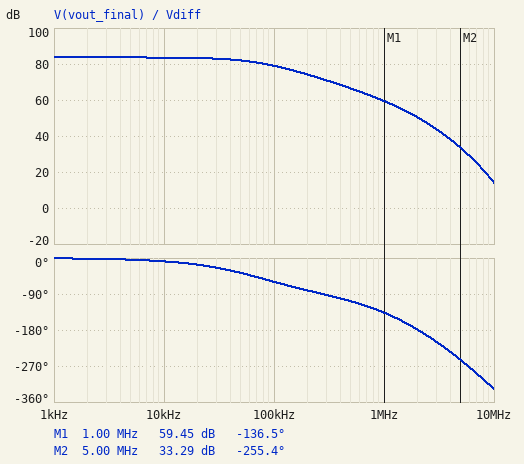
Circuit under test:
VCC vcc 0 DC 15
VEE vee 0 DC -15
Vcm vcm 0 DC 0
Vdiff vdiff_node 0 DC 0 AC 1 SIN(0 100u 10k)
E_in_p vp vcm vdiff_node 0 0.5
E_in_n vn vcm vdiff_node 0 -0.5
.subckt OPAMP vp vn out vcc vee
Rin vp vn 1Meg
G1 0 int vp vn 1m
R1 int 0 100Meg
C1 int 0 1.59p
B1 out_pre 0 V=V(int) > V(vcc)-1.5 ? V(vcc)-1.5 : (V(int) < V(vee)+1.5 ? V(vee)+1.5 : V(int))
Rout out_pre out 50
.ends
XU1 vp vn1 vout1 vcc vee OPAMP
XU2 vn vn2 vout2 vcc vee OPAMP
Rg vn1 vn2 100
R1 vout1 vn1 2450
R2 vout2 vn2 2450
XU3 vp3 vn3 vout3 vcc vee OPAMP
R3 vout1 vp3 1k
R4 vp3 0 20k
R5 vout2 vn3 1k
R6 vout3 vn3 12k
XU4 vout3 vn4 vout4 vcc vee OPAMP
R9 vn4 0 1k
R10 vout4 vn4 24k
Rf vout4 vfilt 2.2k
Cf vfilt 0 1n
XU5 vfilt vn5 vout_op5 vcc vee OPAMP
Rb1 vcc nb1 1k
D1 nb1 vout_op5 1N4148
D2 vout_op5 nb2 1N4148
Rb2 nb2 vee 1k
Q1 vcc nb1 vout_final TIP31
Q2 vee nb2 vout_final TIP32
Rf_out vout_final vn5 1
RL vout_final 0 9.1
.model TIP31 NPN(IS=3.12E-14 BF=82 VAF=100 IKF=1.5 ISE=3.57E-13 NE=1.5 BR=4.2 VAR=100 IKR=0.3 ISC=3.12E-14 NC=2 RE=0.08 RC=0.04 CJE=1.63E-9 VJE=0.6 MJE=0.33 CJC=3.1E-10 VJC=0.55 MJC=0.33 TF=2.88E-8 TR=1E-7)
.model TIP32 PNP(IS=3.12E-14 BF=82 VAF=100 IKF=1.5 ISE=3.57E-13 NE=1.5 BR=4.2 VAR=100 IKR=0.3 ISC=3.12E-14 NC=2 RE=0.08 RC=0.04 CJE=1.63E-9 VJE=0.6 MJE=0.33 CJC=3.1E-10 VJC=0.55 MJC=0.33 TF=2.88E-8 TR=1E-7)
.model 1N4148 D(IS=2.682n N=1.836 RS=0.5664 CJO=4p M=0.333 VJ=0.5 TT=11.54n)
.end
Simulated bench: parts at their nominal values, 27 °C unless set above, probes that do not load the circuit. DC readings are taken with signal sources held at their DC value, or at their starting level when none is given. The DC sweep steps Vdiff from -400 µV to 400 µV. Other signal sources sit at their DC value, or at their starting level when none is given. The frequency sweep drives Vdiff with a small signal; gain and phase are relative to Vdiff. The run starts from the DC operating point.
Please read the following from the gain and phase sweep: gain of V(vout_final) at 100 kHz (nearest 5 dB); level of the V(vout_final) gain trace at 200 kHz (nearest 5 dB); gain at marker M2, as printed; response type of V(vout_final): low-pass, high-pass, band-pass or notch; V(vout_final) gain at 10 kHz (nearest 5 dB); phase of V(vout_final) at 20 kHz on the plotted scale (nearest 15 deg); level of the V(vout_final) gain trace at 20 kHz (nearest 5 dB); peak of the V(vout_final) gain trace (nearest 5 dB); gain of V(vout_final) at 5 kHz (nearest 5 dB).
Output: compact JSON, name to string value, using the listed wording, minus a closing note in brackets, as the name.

{"gain of V(vout_final) at 100 kHz": "80 dB", "level of the V(vout_final) gain trace at 200 kHz": "75 dB", "gain at marker M2, as printed": "33.29 dB", "response type of V(vout_final): low-pass, high-pass, band-pass or notch": "low-pass", "V(vout_final) gain at 10 kHz": "85 dB", "phase of V(vout_final) at 20 kHz on the plotted scale": "-15 deg", "level of the V(vout_final) gain trace at 20 kHz": "85 dB", "peak of the V(vout_final) gain trace": "85 dB", "gain of V(vout_final) at 5 kHz": "85 dB"}
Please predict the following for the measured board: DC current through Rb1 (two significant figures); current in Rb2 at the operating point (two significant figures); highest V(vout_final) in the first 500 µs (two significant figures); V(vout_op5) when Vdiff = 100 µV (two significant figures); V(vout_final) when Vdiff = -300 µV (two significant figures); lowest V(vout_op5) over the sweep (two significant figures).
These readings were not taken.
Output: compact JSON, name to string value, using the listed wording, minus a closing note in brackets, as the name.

{"DC current through Rb1": "14 mA", "current in Rb2 at the operating point": "14 mA", "highest V(vout_final) in the first 500 µs": "1.5 V", "V(vout_op5) when Vdiff = 100 µV": "1.6 V", "V(vout_final) when Vdiff = -300 µV": "-4.6 V", "lowest V(vout_op5) over the sweep": "-12 V"}
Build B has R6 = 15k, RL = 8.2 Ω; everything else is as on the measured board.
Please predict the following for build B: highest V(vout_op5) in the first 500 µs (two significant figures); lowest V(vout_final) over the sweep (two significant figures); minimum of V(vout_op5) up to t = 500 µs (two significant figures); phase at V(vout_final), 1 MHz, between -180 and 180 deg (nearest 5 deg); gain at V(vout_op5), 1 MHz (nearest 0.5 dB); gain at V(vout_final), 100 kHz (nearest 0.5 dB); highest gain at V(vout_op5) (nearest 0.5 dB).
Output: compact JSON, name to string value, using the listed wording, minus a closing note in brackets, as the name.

{"highest V(vout_op5) in the first 500 µs": "1.9 V", "lowest V(vout_final) over the sweep": "-4.9 V", "minimum of V(vout_op5) up to t = 500 µs": "-1.9 V", "phase at V(vout_final), 1 MHz, between -180 and 180 deg": "-140 deg", "gain at V(vout_op5), 1 MHz": "61.5 dB", "gain at V(vout_final), 100 kHz": "81.0 dB", "highest gain at V(vout_op5)": "86.0 dB"}
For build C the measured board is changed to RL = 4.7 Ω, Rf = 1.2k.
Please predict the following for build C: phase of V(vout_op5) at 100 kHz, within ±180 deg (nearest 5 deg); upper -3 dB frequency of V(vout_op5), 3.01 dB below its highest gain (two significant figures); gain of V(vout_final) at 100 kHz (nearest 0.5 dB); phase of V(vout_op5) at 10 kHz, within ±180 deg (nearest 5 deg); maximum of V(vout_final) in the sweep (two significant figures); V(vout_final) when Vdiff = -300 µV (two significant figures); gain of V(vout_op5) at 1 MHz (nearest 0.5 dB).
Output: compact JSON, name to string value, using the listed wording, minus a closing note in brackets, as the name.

{"phase of V(vout_op5) at 100 kHz, within ±180 deg": "-40 deg", "upper -3 dB frequency of V(vout_op5), 3.01 dB below its highest gain": "130 kHz", "gain of V(vout_final) at 100 kHz": "81.5 dB", "phase of V(vout_op5) at 10 kHz, within ±180 deg": "-5 deg", "maximum of V(vout_final) in the sweep": "3.2 V", "V(vout_final) when Vdiff = -300 µV": "-3.2 V", "gain of V(vout_op5) at 1 MHz": "65.5 dB"}
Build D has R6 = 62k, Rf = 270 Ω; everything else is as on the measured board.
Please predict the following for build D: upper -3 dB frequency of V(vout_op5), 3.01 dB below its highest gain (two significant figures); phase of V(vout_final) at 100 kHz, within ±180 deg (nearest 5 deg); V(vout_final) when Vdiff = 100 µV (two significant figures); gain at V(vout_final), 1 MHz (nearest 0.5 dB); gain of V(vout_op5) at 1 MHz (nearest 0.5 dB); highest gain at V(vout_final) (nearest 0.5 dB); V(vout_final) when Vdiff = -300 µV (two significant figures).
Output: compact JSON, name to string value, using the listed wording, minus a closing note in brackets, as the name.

{"upper -3 dB frequency of V(vout_op5), 3.01 dB below its highest gain": "500 kHz", "phase of V(vout_final) at 100 kHz, within ±180 deg": "-20 deg", "V(vout_final) when Vdiff = 100 µV": "5.2 V", "gain at V(vout_final), 1 MHz": "89.0 dB", "gain of V(vout_op5) at 1 MHz": "89.5 dB", "highest gain at V(vout_final)": "97.5 dB", "V(vout_final) when Vdiff = -300 µV": "-5.2 V"}
